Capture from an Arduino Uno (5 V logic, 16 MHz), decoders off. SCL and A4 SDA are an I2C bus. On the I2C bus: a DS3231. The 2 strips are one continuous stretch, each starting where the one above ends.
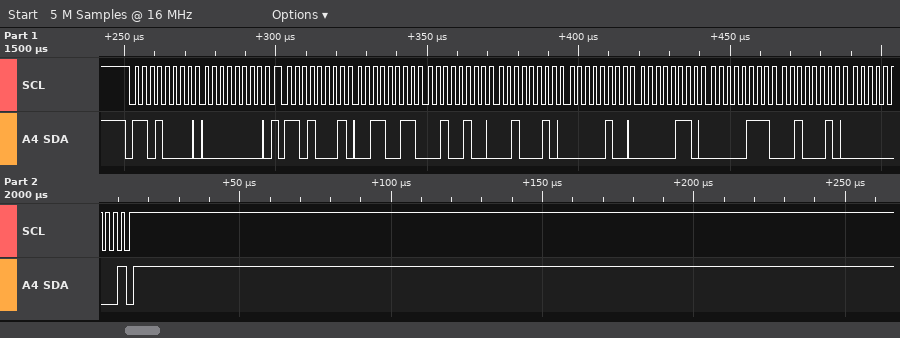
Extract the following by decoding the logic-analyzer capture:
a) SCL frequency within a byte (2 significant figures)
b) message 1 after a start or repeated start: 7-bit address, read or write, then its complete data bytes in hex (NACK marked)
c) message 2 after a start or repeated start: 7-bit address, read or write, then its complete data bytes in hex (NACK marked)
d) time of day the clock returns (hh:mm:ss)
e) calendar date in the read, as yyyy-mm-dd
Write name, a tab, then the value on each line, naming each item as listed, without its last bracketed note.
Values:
SCL frequency within a byte	400 kHz
message 1 after a start or repeated start: 7-bit address, read or write, then its complete data bytes in hex	0x68 write: 00
message 2 after a start or repeated start: 7-bit address, read or write, then its complete data bytes in hex	0x68 read: 33 24 22 04 06 07 22 00 NACK
time of day the clock returns	22:24:33
calendar date in the read, as yyyy-mm-dd	2022-07-06
